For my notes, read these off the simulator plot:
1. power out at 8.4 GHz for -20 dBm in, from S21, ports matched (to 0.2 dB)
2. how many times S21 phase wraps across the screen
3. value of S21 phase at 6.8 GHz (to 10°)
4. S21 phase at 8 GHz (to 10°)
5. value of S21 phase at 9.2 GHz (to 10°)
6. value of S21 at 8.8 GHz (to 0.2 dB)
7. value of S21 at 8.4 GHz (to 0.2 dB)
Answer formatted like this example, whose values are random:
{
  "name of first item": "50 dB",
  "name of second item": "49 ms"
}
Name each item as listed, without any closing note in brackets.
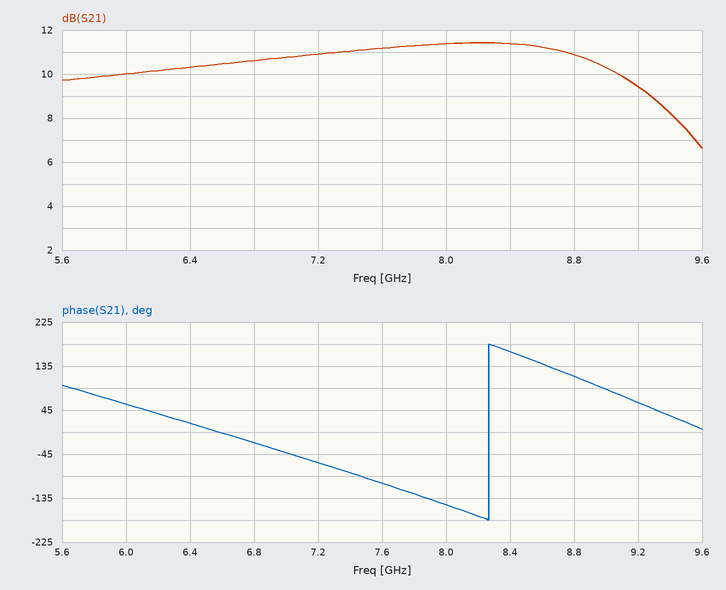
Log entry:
{
  "power out at 8.4 GHz for -20 dBm in, from S21, ports matched": "-8.6 dBm",
  "how many times S21 phase wraps across the screen": "1",
  "value of S21 phase at 6.8 GHz": "-20°",
  "S21 phase at 8 GHz": "-150°",
  "value of S21 phase at 9.2 GHz": "60°",
  "value of S21 at 8.8 GHz": "10.8 dB",
  "value of S21 at 8.4 GHz": "11.4 dB"
}
